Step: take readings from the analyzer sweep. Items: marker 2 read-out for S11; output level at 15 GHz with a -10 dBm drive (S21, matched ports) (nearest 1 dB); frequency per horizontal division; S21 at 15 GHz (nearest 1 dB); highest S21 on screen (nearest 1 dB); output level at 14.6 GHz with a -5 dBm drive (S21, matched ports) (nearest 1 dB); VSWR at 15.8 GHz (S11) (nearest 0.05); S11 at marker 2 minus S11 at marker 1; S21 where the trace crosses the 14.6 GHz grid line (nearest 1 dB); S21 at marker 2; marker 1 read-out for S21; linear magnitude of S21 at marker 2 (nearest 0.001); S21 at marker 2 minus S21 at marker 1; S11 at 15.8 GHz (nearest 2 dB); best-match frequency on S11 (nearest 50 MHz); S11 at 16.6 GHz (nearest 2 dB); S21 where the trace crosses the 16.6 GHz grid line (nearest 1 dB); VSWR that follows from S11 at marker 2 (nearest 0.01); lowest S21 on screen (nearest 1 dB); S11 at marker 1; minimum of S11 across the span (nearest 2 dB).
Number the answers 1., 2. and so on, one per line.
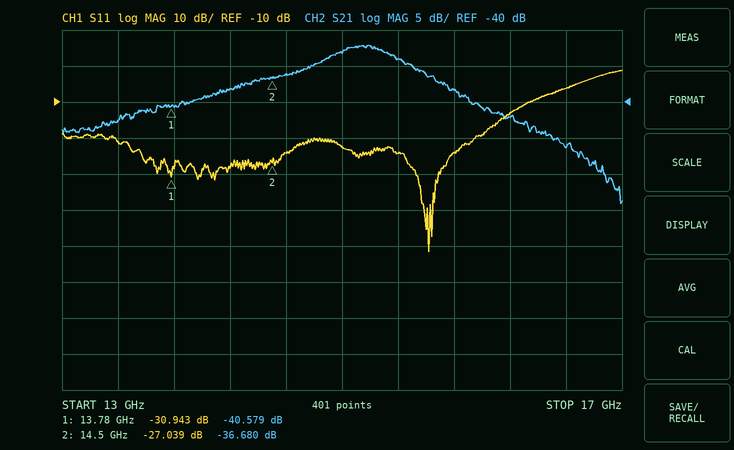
1. -27.039 dB
2. -43 dBm
3. 400 MHz
4. -33 dB
5. -32 dB
6. -41 dBm
7. 1.15
8. 3.904 dB
9. -36 dB
10. -36.680 dB
11. -40.579 dB
12. 0.015
13. 3.899 dB
14. -24 dB
15. 15.60 GHz
16. -6 dB
17. -46 dB
18. 1.09
19. -54 dB
20. -30.943 dB
21. -52 dB
